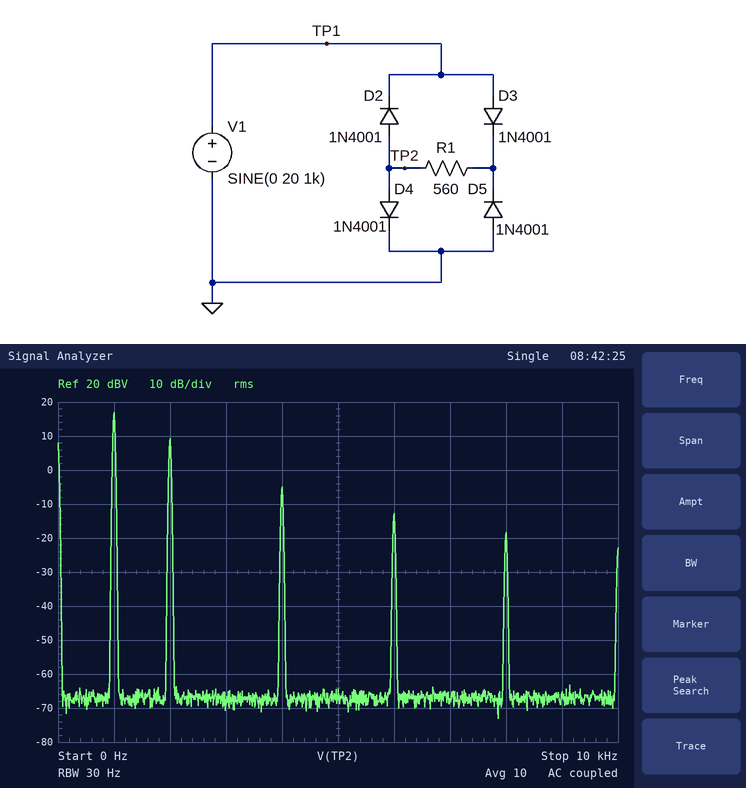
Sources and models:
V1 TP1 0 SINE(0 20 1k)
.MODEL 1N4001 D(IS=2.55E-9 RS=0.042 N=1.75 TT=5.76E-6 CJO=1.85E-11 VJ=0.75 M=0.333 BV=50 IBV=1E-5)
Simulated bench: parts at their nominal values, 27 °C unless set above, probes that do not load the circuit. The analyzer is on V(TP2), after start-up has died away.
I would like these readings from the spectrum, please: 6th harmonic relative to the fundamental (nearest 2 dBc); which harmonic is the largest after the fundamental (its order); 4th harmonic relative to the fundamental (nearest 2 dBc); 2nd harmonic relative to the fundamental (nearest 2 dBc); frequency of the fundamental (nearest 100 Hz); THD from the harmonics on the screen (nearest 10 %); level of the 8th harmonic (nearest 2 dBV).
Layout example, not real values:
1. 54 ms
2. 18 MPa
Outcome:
1. -30 dBc
2. 2
3. -22 dBc
4. -8 dBc
5. 1.0 kHz
6. 40 %
7. -18 dBV
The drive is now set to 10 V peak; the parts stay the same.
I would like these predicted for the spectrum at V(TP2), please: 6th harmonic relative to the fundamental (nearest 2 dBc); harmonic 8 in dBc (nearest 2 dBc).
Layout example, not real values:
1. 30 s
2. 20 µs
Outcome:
1. -32 dBc
2. -40 dBc
